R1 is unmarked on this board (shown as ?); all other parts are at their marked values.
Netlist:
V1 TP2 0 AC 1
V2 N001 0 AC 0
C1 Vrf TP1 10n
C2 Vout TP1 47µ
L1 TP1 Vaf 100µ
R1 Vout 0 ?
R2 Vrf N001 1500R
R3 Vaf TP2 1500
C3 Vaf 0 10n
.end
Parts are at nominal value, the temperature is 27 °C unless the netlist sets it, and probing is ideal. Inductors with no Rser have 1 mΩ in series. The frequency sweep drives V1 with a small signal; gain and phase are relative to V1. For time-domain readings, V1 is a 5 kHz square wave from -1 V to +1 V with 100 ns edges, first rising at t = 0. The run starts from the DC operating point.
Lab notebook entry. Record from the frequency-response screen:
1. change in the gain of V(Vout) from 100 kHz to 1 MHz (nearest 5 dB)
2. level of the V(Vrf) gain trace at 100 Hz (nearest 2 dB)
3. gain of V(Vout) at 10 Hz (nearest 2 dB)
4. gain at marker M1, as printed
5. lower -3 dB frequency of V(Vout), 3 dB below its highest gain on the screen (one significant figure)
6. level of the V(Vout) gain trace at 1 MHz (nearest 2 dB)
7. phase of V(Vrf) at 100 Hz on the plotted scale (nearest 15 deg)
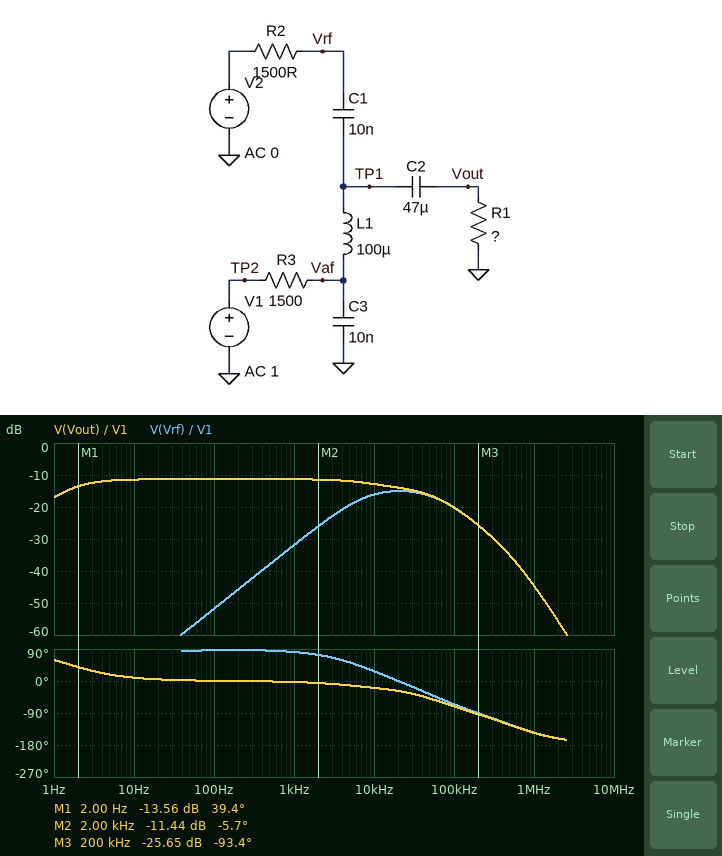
-25 dB
-52 dB
-12 dB
-13.56 dB
2 Hz
-44 dB
90 deg
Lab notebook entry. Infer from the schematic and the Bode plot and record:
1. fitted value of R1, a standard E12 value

560 Ω
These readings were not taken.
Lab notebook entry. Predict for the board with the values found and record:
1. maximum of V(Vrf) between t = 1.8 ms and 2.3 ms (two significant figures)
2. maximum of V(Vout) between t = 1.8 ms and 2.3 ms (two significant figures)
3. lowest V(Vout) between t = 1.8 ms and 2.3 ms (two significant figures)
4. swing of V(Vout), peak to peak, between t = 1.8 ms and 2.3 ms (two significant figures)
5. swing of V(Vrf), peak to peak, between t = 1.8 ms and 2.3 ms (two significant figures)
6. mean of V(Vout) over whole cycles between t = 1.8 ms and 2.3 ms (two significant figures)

290 mV
540 mV
-5.0 mV
540 mV
580 mV
270 mV
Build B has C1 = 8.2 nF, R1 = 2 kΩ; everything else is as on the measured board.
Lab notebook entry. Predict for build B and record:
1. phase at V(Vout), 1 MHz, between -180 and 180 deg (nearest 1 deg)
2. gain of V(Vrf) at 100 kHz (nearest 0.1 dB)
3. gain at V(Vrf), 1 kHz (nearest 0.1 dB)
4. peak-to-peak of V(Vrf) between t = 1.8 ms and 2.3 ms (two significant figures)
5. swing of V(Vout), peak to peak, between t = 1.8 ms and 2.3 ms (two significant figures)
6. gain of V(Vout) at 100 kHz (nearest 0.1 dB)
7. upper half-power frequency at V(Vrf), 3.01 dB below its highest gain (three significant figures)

-125 deg
-19.9 dB
-27.2 dB
800 mV
1.1 V
-19.8 dB
47.9 kHz
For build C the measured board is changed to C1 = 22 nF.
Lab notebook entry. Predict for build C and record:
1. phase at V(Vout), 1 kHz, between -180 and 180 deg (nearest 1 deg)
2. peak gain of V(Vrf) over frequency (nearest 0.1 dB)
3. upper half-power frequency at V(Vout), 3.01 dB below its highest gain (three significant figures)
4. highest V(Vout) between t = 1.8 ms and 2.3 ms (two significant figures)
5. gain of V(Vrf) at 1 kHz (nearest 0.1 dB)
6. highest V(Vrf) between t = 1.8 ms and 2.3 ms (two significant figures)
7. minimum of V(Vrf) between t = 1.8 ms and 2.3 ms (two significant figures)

-4 deg
-14.2 dB
24.4 kHz
530 mV
-25.3 dB
310 mV
-310 mV
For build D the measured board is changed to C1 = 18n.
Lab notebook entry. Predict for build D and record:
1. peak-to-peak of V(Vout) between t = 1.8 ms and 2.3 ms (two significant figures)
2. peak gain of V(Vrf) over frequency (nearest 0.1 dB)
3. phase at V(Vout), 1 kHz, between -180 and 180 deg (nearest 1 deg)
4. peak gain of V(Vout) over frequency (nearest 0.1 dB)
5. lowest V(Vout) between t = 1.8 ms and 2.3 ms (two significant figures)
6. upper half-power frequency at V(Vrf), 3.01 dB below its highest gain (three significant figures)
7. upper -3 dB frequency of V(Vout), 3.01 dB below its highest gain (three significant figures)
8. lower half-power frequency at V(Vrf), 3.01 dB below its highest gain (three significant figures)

530 mV
-14.3 dB
-4 deg
-11.3 dB
1.7 mV
62.6 kHz
24.3 kHz
3.91 kHz
